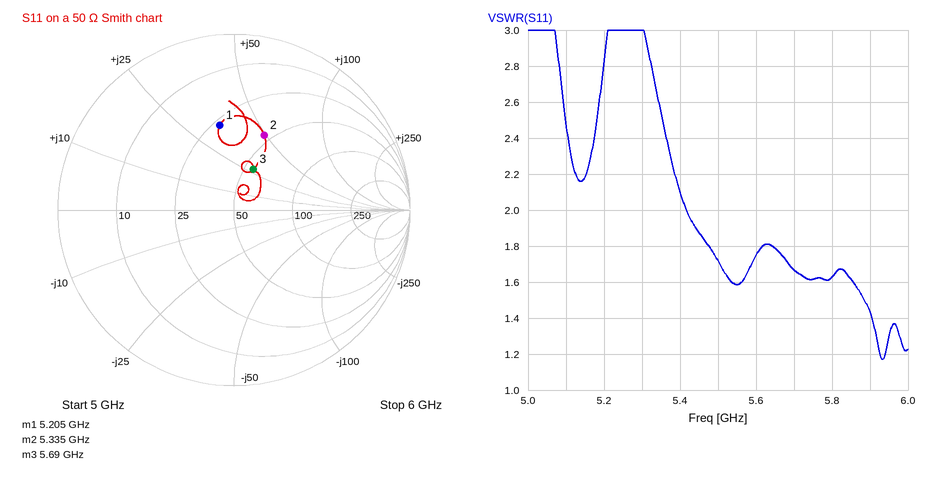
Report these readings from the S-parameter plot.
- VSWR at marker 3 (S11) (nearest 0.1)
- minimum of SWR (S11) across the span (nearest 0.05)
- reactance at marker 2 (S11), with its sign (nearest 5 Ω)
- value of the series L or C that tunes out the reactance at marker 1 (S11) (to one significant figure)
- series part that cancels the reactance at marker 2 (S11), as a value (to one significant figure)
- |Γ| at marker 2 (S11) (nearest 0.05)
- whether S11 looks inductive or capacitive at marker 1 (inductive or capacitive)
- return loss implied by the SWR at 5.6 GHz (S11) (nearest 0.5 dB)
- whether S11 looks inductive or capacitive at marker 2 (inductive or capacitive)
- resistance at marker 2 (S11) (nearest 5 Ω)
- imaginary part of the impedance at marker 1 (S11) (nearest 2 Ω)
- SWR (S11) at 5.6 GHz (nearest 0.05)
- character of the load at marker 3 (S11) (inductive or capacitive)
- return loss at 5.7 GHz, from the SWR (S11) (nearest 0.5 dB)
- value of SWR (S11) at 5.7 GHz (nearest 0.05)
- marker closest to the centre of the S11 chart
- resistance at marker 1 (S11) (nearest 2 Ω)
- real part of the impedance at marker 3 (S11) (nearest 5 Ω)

1.7
1.15
+50 Ω
900 fF
600 fF
0.45
inductive
11.5 dB
inductive
45 Ω
+34 Ω
1.75
inductive
12.0 dB
1.65
marker 3
28 Ω
55 Ω
